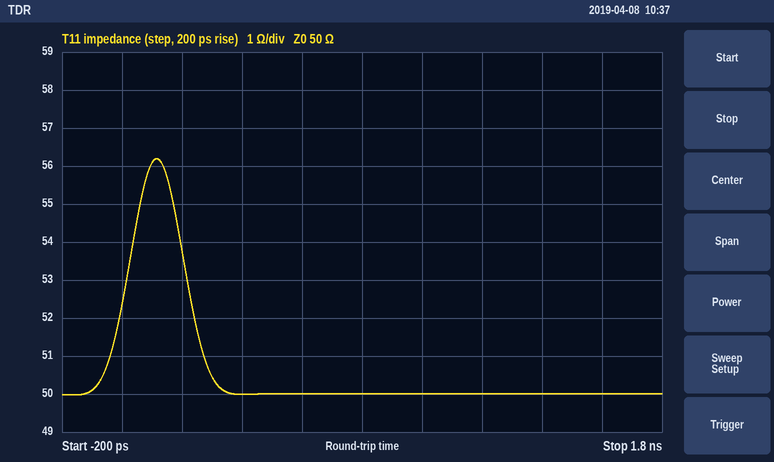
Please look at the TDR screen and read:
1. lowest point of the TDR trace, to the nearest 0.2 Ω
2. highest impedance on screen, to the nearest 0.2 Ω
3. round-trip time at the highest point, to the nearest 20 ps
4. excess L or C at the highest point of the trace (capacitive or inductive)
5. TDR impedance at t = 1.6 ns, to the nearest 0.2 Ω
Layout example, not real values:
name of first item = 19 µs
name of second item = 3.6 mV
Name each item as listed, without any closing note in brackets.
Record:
lowest point of the TDR trace, to the nearest 0.2 Ω = 50.0 Ω
highest impedance on screen, to the nearest 0.2 Ω = 56.2 Ω
round-trip time at the highest point, to the nearest 20 ps = 120 ps
excess L or C at the highest point of the trace = inductive
TDR impedance at t = 1.6 ns, to the nearest 0.2 Ω = 50.0 Ω
